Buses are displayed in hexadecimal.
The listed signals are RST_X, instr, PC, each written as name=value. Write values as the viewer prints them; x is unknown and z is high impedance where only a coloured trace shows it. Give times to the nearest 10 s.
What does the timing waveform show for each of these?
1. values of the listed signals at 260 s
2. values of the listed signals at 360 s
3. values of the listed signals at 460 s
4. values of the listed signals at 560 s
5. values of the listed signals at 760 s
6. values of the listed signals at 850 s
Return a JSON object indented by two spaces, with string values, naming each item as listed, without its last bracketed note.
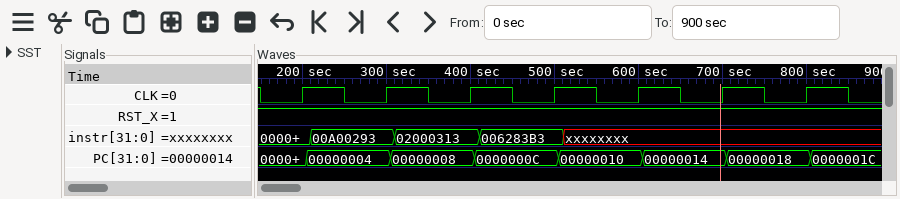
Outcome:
{
  "values of the listed signals at 260 s": "RST_X=1, instr=00A00293, PC=00000004",
  "values of the listed signals at 360 s": "RST_X=1, instr=02000313, PC=00000008",
  "values of the listed signals at 460 s": "RST_X=1, instr=006283B3, PC=0000000C",
  "values of the listed signals at 560 s": "RST_X=1, instr=xxxxxxxx, PC=00000010",
  "values of the listed signals at 760 s": "RST_X=1, instr=xxxxxxxx, PC=00000018",
  "values of the listed signals at 850 s": "RST_X=1, instr=xxxxxxxx, PC=0000001C"
}
